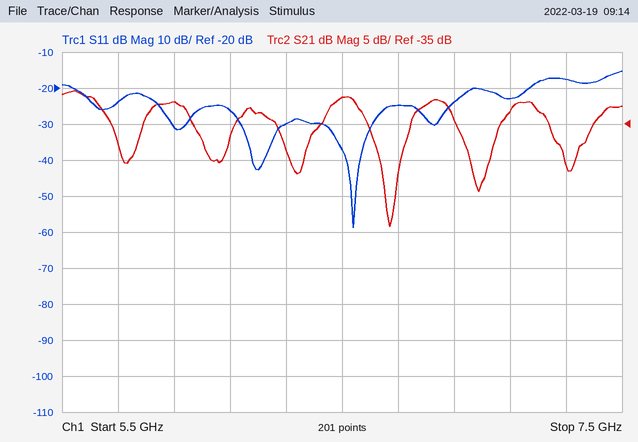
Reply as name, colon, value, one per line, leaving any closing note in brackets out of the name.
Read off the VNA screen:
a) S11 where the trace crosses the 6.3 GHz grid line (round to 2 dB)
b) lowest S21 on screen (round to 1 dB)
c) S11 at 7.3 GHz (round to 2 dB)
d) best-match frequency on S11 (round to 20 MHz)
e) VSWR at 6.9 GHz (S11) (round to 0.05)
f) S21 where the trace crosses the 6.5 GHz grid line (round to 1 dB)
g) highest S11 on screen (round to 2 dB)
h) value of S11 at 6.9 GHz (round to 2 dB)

S11 where the trace crosses the 6.3 GHz grid line: -30 dB
lowest S21 on screen: -49 dB
S11 at 7.3 GHz: -18 dB
best-match frequency on S11: 6.54 GHz
VSWR at 6.9 GHz (S11): 1.15
S21 where the trace crosses the 6.5 GHz grid line: -31 dB
highest S11 on screen: -16 dB
value of S11 at 6.9 GHz: -24 dB
